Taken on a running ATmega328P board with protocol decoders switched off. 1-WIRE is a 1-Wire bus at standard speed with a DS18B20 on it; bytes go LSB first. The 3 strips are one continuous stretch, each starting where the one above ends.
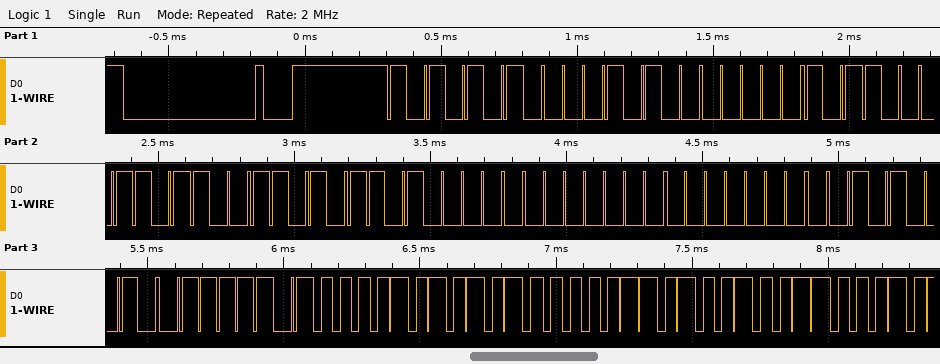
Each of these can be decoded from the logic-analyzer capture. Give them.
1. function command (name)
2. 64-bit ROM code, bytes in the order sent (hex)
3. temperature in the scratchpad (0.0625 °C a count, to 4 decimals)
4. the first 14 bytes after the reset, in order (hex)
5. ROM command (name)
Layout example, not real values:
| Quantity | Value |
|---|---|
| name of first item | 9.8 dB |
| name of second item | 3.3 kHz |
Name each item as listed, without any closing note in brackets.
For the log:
| Quantity | Value |
|---|---|
| function command | Read Scratchpad |
| 64-bit ROM code, bytes in the order sent | 28 A0 B1 59 0B 00 00 4A |
| temperature in the scratchpad | 85.0000 °C |
| the first 14 bytes after the reset, in order | 55 28 A0 B1 59 0B 00 00 4A BE 50 05 4B 46 |
| ROM command | Match ROM |
